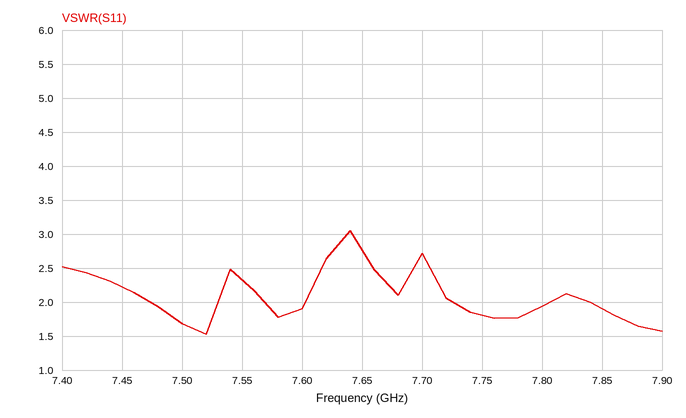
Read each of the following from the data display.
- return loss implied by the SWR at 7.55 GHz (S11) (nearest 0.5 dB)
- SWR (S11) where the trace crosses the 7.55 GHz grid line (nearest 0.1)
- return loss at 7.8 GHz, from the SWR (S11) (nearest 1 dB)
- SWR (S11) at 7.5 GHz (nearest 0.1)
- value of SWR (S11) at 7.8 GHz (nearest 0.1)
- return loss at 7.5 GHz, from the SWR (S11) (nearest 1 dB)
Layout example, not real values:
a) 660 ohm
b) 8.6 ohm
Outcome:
a) 8.0 dB
b) 2.3
c) 10 dB
d) 1.7
e) 1.9
f) 12 dB
